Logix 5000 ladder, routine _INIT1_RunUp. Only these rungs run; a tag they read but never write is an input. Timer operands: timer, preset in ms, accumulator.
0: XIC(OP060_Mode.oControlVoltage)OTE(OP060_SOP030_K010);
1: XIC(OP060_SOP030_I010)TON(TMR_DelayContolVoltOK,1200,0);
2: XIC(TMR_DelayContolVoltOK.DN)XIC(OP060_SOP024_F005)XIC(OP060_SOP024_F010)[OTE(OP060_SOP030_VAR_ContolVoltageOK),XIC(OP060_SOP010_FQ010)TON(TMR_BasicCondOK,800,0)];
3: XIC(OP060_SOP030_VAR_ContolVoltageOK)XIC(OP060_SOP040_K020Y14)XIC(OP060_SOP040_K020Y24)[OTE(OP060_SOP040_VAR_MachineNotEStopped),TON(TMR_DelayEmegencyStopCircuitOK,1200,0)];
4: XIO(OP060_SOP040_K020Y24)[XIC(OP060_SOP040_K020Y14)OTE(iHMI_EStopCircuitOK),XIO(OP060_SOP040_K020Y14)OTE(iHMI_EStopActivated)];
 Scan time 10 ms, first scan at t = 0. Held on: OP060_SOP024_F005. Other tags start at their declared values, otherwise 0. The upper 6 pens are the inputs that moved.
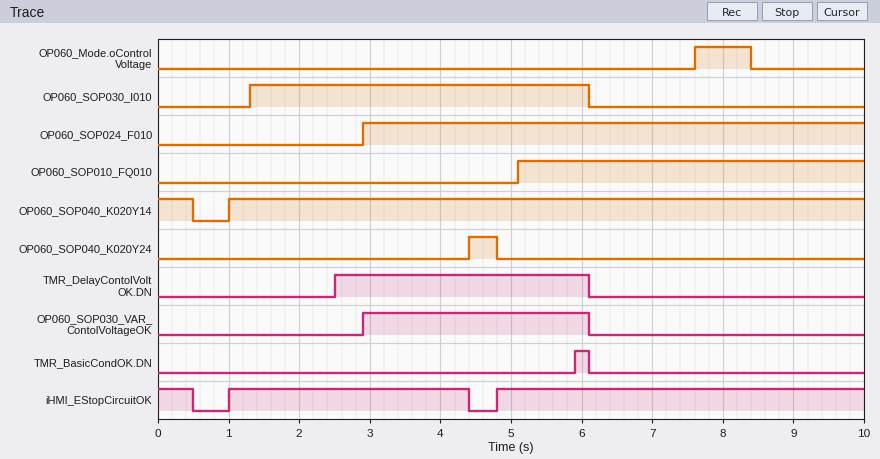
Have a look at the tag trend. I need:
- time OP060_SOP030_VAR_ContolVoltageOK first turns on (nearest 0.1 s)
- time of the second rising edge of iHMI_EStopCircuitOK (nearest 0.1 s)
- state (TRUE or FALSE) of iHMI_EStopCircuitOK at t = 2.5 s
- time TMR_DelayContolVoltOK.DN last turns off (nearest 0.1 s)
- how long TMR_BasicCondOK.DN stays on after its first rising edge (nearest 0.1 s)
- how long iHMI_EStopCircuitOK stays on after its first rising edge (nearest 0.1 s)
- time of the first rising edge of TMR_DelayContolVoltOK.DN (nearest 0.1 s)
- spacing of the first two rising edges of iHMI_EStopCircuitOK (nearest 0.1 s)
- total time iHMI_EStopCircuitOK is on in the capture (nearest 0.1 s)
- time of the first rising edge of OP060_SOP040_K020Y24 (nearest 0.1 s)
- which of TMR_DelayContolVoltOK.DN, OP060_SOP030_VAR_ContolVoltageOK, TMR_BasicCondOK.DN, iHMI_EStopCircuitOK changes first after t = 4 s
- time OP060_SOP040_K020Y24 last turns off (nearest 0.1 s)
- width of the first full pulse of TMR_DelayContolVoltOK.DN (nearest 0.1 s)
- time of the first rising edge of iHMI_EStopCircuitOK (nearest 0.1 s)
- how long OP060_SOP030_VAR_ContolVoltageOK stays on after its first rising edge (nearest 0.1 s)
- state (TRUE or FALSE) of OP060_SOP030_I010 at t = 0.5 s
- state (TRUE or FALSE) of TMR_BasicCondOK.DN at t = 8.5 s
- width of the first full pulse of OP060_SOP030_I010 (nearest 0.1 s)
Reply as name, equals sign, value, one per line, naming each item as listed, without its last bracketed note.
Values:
time OP060_SOP030_VAR_ContolVoltageOK first turns on = 2.9 s
time of the second rising edge of iHMI_EStopCircuitOK = 4.8 s
state (TRUE or FALSE) of iHMI_EStopCircuitOK at t = 2.5 s = TRUE
time TMR_DelayContolVoltOK.DN last turns off = 6.1 s
how long TMR_BasicCondOK.DN stays on after its first rising edge = 0.2 s
how long iHMI_EStopCircuitOK stays on after its first rising edge = 3.4 s
time of the first rising edge of TMR_DelayContolVoltOK.DN = 2.5 s
spacing of the first two rising edges of iHMI_EStopCircuitOK = 3.8 s
total time iHMI_EStopCircuitOK is on in the capture = 9.1 s
time of the first rising edge of OP060_SOP040_K020Y24 = 4.4 s
which of TMR_DelayContolVoltOK.DN, OP060_SOP030_VAR_ContolVoltageOK, TMR_BasicCondOK.DN, iHMI_EStopCircuitOK changes first after t = 4 s = iHMI_EStopCircuitOK
time OP060_SOP040_K020Y24 last turns off = 4.8 s
width of the first full pulse of TMR_DelayContolVoltOK.DN = 3.6 s
time of the first rising edge of iHMI_EStopCircuitOK = 1.0 s
how long OP060_SOP030_VAR_ContolVoltageOK stays on after its first rising edge = 3.2 s
state (TRUE or FALSE) of OP060_SOP030_I010 at t = 0.5 s = FALSE
state (TRUE or FALSE) of TMR_BasicCondOK.DN at t = 8.5 s = FALSE
width of the first full pulse of OP060_SOP030_I010 = 4.8 s
